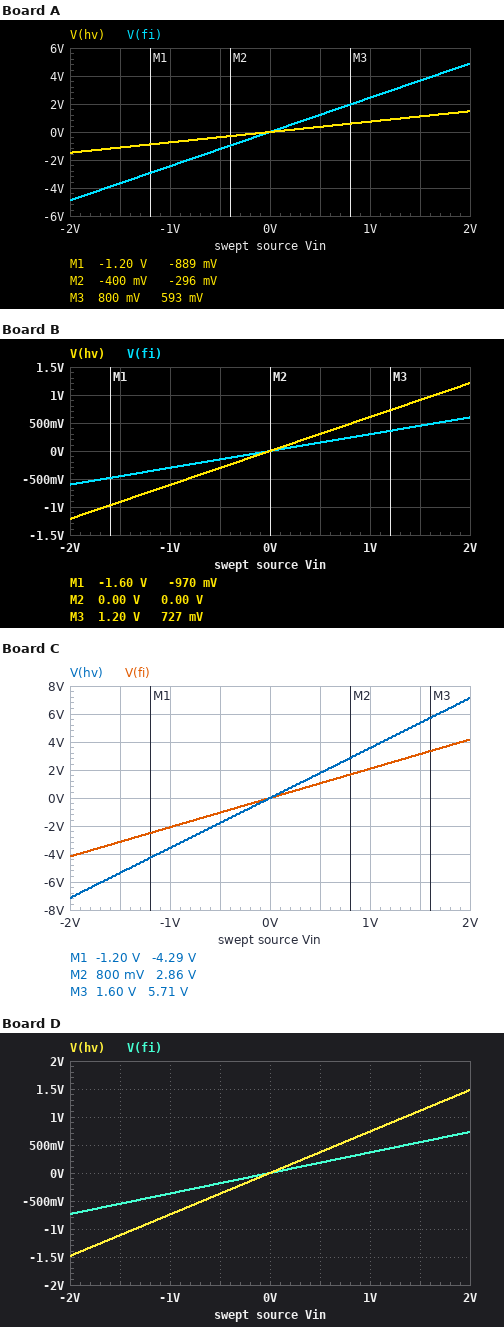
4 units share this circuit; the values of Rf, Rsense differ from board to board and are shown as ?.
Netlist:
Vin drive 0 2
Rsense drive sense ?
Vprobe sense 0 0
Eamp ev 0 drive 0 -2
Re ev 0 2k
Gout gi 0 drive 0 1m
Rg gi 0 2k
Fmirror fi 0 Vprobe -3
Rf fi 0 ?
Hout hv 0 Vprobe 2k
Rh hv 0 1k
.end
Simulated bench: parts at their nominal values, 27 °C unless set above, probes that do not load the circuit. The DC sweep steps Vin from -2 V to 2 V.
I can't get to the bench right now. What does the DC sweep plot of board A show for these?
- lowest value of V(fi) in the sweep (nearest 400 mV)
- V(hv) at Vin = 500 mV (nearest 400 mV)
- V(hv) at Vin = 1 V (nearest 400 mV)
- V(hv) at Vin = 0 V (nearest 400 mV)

-4.8 V
400 mV
800 mV
0 V
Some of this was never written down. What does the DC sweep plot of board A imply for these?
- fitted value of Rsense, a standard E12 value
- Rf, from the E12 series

2.7 kΩ
2.2 kΩ
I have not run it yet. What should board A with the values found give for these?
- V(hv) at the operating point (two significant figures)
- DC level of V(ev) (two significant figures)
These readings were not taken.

1.5 V
-4.0 V
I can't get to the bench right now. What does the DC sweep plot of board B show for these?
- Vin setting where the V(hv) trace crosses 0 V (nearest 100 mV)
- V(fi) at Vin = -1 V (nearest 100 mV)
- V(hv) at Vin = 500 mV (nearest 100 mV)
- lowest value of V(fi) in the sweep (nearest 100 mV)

0 V
-300 mV
300 mV
-600 mV
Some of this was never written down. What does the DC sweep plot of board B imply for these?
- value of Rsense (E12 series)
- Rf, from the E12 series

3.3 kΩ
330 Ω
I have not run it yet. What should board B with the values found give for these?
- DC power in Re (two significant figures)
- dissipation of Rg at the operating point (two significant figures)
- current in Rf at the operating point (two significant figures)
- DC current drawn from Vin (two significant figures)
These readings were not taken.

8.0 mW
8.0 mW
1.8 mA
610 µA
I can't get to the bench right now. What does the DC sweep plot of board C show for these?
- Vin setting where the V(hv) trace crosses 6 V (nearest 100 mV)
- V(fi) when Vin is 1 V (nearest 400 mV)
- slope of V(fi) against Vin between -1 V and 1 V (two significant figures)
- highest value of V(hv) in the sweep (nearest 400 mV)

1.7 V
2.0 V
2.1 V/V
7.2 V
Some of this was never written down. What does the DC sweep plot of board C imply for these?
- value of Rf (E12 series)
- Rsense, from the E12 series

390 Ω
560 Ω
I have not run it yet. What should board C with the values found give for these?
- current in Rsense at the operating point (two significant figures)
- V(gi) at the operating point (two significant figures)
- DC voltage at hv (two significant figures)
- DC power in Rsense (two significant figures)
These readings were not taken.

3.6 mA
-4.0 V
7.1 V
7.1 mW
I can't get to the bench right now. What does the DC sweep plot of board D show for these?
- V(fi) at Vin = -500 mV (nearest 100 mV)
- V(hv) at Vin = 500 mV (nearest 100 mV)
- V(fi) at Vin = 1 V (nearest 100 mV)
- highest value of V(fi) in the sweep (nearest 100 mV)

-200 mV
400 mV
400 mV
700 mV
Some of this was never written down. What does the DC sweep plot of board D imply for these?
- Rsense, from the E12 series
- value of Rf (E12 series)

2.7 kΩ
330 Ω
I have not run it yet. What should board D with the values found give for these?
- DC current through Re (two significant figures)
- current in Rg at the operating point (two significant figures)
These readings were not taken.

2.0 mA
2.0 mA
